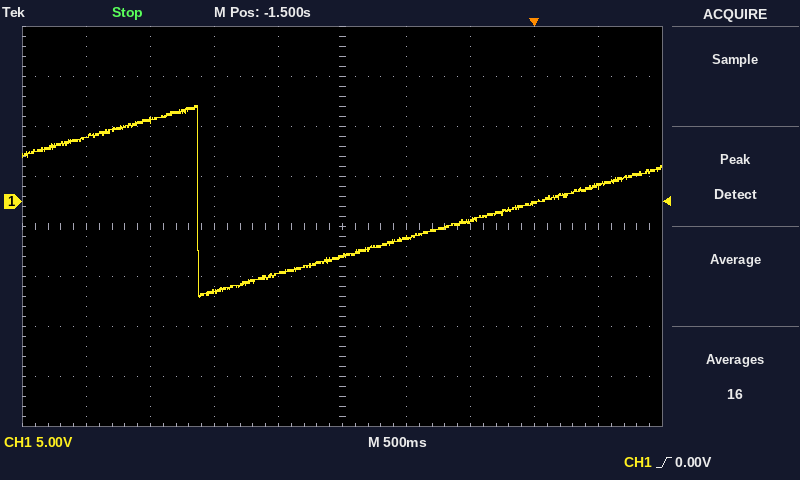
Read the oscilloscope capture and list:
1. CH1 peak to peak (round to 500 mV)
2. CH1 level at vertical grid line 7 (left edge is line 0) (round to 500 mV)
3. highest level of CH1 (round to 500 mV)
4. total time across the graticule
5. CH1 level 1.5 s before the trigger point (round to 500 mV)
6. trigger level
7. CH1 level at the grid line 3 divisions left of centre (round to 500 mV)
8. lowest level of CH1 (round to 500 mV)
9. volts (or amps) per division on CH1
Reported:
19.0 V
-2.0 V
9.5 V
5 s
-5.5 V
0.00 V
8.0 V
-9.5 V
5 V
